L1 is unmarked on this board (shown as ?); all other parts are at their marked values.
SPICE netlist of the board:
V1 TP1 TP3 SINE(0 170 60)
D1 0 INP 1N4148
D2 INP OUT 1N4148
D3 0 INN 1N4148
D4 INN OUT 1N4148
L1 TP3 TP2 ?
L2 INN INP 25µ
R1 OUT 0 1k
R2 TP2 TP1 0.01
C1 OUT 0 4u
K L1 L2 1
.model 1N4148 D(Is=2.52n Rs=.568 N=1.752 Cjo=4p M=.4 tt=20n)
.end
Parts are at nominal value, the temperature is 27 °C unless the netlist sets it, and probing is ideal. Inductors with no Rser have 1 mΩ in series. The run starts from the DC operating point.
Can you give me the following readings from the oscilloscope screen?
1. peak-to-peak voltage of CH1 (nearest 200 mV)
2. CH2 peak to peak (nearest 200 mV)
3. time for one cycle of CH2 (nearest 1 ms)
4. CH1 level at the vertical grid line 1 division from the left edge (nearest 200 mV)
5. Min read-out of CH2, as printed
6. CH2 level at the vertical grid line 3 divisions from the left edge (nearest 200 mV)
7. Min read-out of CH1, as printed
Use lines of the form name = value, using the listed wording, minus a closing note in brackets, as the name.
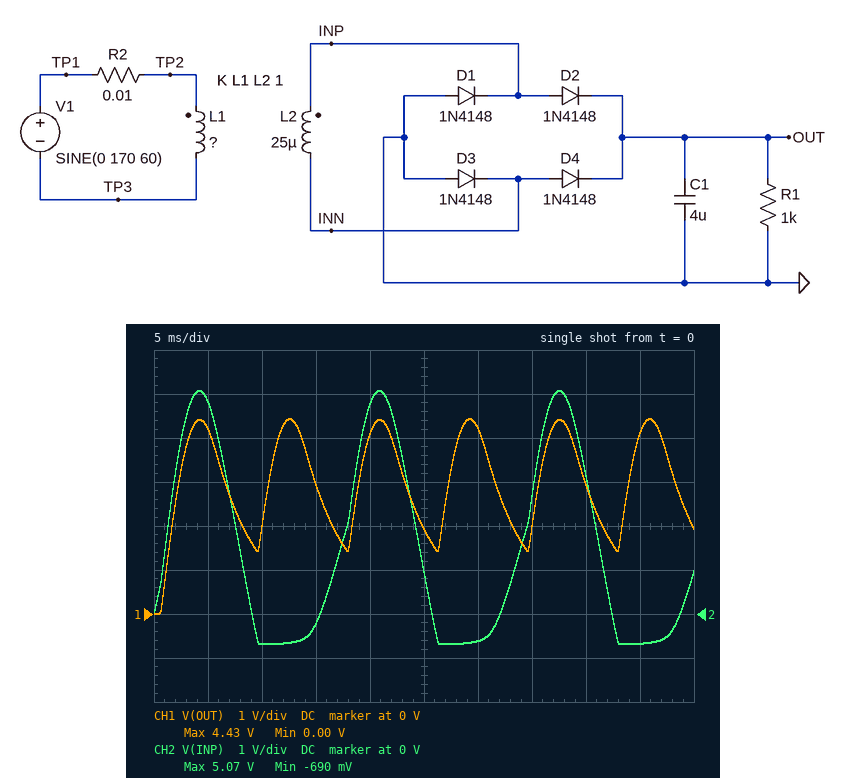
peak-to-peak voltage of CH1 = 4.4 V
CH2 peak to peak = 5.8 V
time for one cycle of CH2 = 17 ms
CH1 level at the vertical grid line 1 division from the left edge = 4.2 V
Min read-out of CH2, as printed = -690 mV
CH2 level at the vertical grid line 3 divisions from the left edge = -200 mV
Min read-out of CH1, as printed = 0.00 V
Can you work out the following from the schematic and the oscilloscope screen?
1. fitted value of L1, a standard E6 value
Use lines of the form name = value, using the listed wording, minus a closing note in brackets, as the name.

fitted value of L1, a standard E6 value = 22 mH
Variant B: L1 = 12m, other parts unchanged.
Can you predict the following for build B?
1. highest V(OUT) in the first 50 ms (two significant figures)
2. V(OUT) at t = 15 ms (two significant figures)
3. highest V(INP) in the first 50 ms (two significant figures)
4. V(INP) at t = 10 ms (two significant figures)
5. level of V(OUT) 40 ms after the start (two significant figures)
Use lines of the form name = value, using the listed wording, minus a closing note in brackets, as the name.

highest V(OUT) in the first 50 ms = 6.4 V
V(OUT) at t = 15 ms = 4.3 V
highest V(INP) in the first 50 ms = 7.1 V
V(INP) at t = 10 ms = -710 mV
level of V(OUT) 40 ms after the start = 4.2 V
